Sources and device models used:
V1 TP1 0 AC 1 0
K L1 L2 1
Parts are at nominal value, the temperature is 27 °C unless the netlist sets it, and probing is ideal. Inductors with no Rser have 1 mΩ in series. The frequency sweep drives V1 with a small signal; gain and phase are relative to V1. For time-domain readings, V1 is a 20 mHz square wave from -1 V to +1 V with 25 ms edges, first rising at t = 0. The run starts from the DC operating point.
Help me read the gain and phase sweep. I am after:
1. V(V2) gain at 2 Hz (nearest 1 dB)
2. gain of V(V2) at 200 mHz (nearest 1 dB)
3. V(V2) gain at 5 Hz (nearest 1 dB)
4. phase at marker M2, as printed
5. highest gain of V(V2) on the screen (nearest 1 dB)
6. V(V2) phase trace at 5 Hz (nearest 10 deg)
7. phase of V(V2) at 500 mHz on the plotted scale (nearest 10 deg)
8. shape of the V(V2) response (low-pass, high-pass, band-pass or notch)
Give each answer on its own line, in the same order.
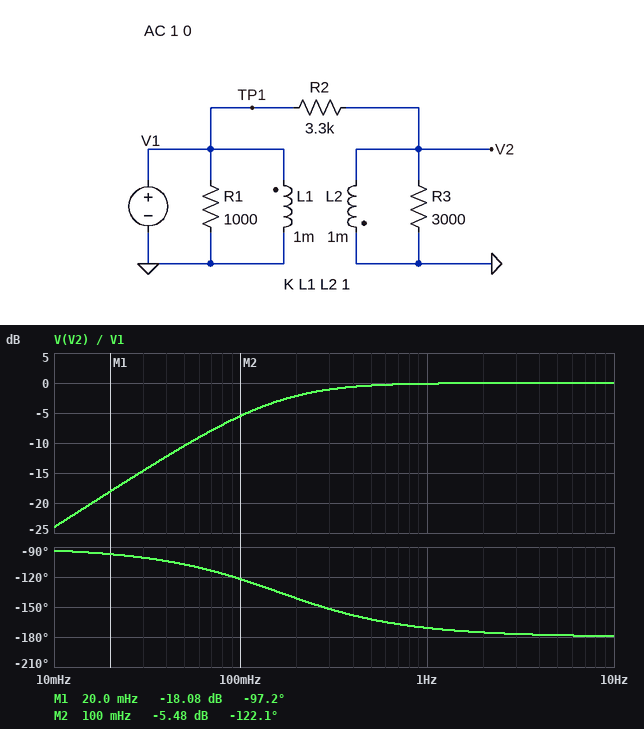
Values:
0 dB
-2 dB
0 dB
-122.1 deg
0 dB
-180 deg
-160 deg
high-pass
